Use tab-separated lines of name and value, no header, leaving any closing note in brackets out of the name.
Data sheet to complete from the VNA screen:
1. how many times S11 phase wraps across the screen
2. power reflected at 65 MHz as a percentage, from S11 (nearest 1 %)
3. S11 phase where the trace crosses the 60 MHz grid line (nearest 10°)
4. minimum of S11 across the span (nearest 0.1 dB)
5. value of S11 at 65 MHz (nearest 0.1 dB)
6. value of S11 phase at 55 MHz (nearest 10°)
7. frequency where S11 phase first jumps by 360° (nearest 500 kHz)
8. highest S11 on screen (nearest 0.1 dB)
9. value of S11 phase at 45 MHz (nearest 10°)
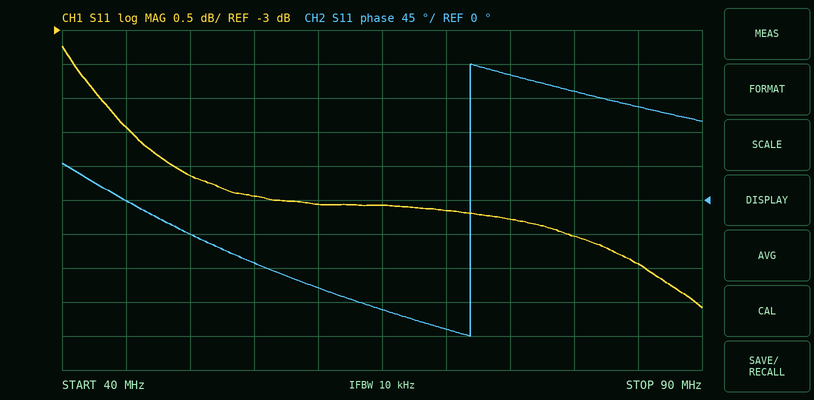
how many times S11 phase wraps across the screen	1
power reflected at 65 MHz as a percentage, from S11	28 %
S11 phase where the trace crosses the 60 MHz grid line	-120°
minimum of S11 across the span	-7.1 dB
value of S11 at 65 MHz	-5.6 dB
value of S11 phase at 55 MHz	-80°
frequency where S11 phase first jumps by 360°	72.0 MHz
highest S11 on screen	-3.2 dB
value of S11 phase at 45 MHz	0°
